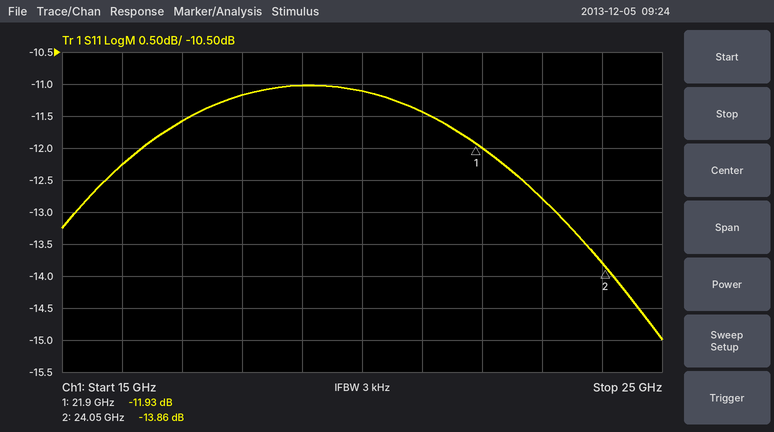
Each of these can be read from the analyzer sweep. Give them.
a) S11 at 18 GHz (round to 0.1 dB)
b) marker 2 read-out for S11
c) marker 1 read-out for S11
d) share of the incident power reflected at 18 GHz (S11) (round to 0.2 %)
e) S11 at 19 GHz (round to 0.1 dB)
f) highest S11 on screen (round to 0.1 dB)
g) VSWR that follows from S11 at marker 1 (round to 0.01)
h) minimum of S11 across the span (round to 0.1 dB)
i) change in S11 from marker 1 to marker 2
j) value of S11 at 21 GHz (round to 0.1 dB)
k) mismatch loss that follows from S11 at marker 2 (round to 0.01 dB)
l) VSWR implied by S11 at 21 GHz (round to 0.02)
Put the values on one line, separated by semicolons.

-11.2 dB; -13.86 dB; -11.93 dB; 7.6 %; -11.0 dB; -11.0 dB; 1.68; -15.0 dB; -1.93 dB; -11.4 dB; 0.18 dB; 1.74
